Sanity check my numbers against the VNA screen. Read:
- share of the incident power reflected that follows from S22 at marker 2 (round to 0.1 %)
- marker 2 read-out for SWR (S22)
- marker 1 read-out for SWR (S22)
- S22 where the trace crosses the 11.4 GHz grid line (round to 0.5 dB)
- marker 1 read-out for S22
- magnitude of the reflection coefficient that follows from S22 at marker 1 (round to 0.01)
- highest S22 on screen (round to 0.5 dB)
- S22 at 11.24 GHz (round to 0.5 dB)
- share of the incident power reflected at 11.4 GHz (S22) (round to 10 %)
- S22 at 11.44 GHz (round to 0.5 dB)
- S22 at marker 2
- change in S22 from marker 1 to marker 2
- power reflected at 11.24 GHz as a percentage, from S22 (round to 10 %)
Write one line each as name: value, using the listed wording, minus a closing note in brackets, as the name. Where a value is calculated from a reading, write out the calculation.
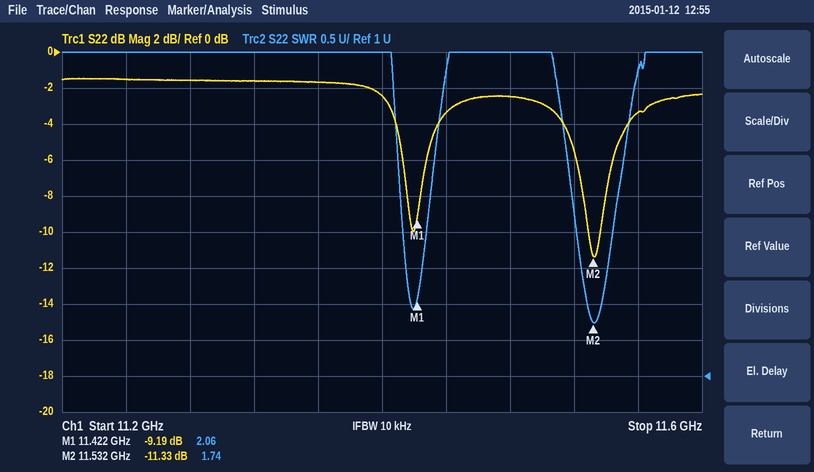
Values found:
share of the incident power reflected that follows from S22 at marker 2: 10^(-11.33/10) ≈ 7.4 %
marker 2 read-out for SWR: 1.74
marker 1 read-out for SWR: 2.06
S22 where the trace crosses the 11.4 GHz grid line: -2.5 dB
marker 1 read-out for S22: -9.19 dB
magnitude of the reflection coefficient that follows from S22 at marker 1: 10^(-9.19/20) ≈ 0.35
highest S22 on screen: -1.5 dB
S22 at 11.24 GHz: -1.5 dB
share of the incident power reflected at 11.4 GHz (S22): 10^(-2.5/10) ≈ 56.2 %, so 60 % to the nearest 10 %
S22 at 11.44 GHz: -3.5 dB
S22 at marker 2: -11.33 dB
change in S22 from marker 1 to marker 2: -11.33 − (-9.19) = -2.14 dB
power reflected at 11.24 GHz as a percentage, from S22: 10^(-1.5/10) ≈ 70.8 %, so 70 % to the nearest 10 %
